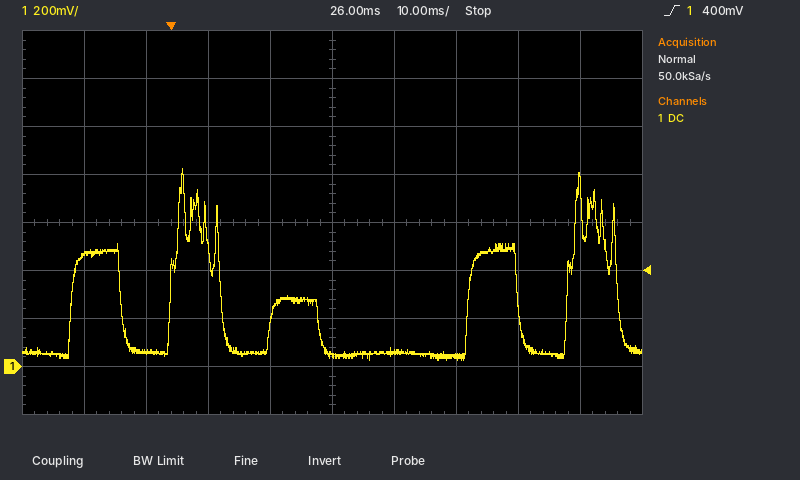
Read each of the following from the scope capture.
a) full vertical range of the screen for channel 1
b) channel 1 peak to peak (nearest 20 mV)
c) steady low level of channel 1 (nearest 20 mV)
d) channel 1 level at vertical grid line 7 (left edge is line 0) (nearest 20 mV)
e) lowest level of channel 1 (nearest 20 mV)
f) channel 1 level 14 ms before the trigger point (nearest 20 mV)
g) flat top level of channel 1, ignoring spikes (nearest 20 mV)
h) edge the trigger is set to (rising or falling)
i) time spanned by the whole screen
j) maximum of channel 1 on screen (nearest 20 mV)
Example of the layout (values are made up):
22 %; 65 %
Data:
1.6 V; 800 mV; 60 mV; 40 mV; 20 mV; 460 mV; 480 mV; rising; 100 ms; 820 mV
